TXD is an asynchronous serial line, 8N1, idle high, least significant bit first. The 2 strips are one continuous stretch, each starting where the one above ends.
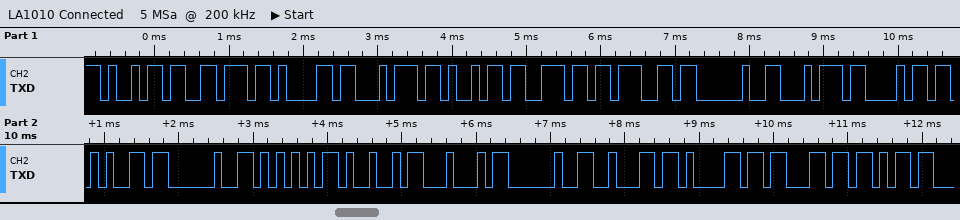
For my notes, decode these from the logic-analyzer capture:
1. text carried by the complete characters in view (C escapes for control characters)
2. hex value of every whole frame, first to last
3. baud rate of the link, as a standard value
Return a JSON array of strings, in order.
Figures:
["\"ivating the UID back\"", "69 76 61 74 69 6E 67 20 74 68 65 20 55 49 44 20 62 61 63 6B", "9600 baud"]
